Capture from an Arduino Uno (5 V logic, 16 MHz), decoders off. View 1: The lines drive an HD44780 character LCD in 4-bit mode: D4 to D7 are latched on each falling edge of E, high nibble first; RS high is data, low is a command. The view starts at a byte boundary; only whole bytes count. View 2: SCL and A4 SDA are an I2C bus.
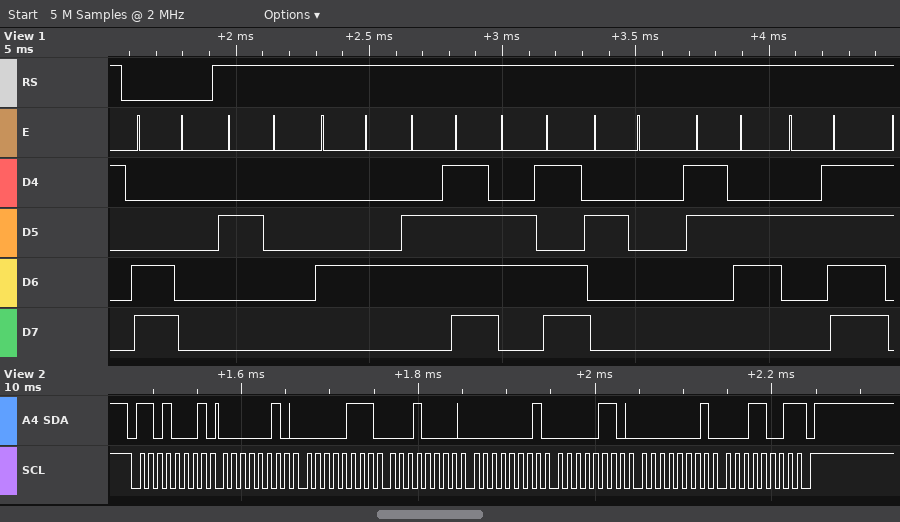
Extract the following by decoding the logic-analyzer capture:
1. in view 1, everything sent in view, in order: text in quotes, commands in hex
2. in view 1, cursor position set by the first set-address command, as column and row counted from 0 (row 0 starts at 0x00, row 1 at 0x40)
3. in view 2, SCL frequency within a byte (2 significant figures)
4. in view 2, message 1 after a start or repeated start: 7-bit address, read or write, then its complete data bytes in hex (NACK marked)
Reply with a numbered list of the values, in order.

1. 0xC0 " Dom 6/"
2. column 0, row 1
3. 100 kHz
4. 0x68 read: 02 07 10 01 06 01 19 NACK
